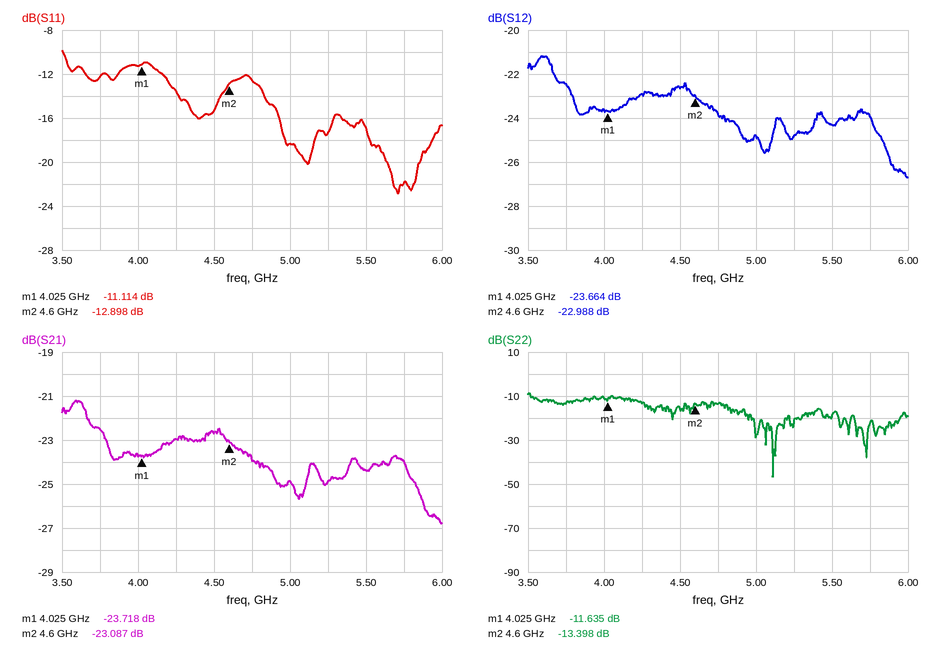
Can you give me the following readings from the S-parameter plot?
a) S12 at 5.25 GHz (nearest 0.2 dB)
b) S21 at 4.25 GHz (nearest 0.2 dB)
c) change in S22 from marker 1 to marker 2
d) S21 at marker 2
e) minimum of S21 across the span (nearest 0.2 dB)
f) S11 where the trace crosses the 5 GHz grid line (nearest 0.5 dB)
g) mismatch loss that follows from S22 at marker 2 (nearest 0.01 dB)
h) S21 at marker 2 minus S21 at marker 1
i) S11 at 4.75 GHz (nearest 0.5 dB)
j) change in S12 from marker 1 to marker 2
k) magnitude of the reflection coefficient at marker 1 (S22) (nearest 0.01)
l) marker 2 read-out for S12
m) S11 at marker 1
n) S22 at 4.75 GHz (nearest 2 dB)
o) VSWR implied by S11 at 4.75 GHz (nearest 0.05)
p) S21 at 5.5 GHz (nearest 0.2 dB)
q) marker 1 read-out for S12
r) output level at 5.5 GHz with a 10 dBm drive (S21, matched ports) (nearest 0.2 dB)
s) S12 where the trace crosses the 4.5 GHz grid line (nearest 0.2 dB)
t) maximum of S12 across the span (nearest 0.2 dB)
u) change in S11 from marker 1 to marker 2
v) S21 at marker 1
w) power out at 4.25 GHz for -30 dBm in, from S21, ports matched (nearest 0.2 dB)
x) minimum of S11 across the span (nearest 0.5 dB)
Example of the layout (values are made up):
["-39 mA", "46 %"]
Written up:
["-24.8 dB", "-23.0 dB", "-1.763 dB", "-23.087 dB", "-26.8 dB", "-18.5 dB", "0.20 dB", "0.631 dB", "-12.5 dB", "0.676 dB", "0.26", "-22.988 dB", "-11.114 dB", "-14 dB", "1.60", "-24.4 dB", "-23.664 dB", "-14.4 dBm", "-22.6 dB", "-21.2 dB", "-1.784 dB", "-23.718 dB", "-53.0 dBm", "-23.0 dB"]
